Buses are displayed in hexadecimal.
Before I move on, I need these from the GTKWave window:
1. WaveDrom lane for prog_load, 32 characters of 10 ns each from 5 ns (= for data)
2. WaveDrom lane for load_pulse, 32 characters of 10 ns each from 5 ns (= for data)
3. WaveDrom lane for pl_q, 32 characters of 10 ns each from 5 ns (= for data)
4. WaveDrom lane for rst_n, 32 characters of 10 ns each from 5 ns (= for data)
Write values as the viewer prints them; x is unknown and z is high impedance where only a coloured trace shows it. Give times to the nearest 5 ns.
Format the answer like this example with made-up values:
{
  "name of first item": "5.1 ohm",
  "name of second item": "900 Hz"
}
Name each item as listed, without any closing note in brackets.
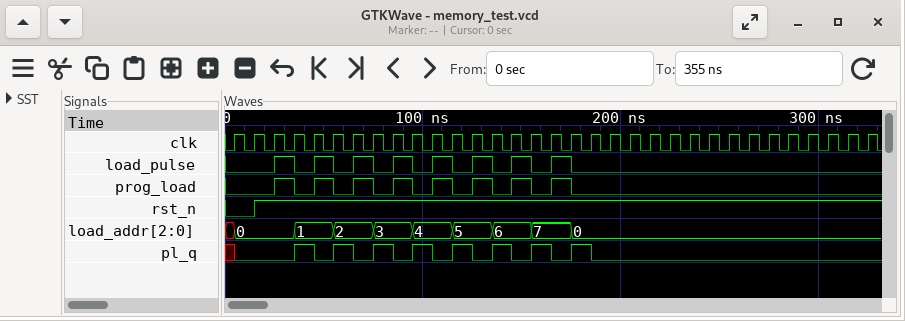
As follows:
{
  "WaveDrom lane for prog_load, 32 characters of 10 ns each from 5 ns": "{name: 'prog_load', wave: '0.1010101010101010..............'}",
  "WaveDrom lane for load_pulse, 32 characters of 10 ns each from 5 ns": "{name: 'load_pulse', wave: '0.1010101010101010..............'}",
  "WaveDrom lane for pl_q, 32 characters of 10 ns each from 5 ns": "{name: 'pl_q', wave: '0..1010101010101010.............'}",
  "WaveDrom lane for rst_n, 32 characters of 10 ns each from 5 ns": "{name: 'rst_n', wave: '01..............................'}"
}
